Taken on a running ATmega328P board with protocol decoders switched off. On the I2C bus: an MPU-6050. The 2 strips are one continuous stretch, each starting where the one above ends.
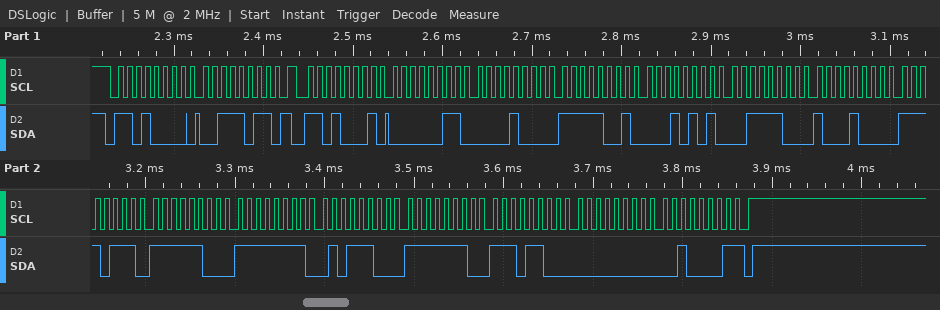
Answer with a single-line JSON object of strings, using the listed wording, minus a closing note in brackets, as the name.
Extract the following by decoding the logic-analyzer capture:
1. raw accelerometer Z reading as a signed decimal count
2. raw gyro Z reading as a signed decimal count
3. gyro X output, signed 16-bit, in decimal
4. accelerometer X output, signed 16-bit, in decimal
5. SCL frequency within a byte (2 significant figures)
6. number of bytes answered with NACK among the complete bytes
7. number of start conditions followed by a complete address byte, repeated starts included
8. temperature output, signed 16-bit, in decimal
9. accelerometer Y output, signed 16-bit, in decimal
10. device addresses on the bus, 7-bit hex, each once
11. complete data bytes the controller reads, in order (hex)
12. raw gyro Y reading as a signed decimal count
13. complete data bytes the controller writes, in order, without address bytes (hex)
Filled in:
{"raw accelerometer Z reading as a signed decimal count": "15496", "raw gyro Z reading as a signed decimal count": "33", "gyro X output, signed 16-bit, in decimal": "-164", "accelerometer X output, signed 16-bit, in decimal": "776", "SCL frequency within a byte": "100 kHz", "number of bytes answered with NACK among the complete bytes": "1", "number of start conditions followed by a complete address byte, repeated starts included": "2", "temperature output, signed 16-bit, in decimal": "-2052", "accelerometer Y output, signed 16-bit, in decimal": "-1771", "device addresses on the bus, 7-bit hex, each once": "0x68", "complete data bytes the controller reads, in order": "03 08 F9 15 3C 88 F7 FC FF 5C FE EC 00 21", "raw gyro Y reading as a signed decimal count": "-276", "complete data bytes the controller writes, in order, without address bytes": "3B"}
